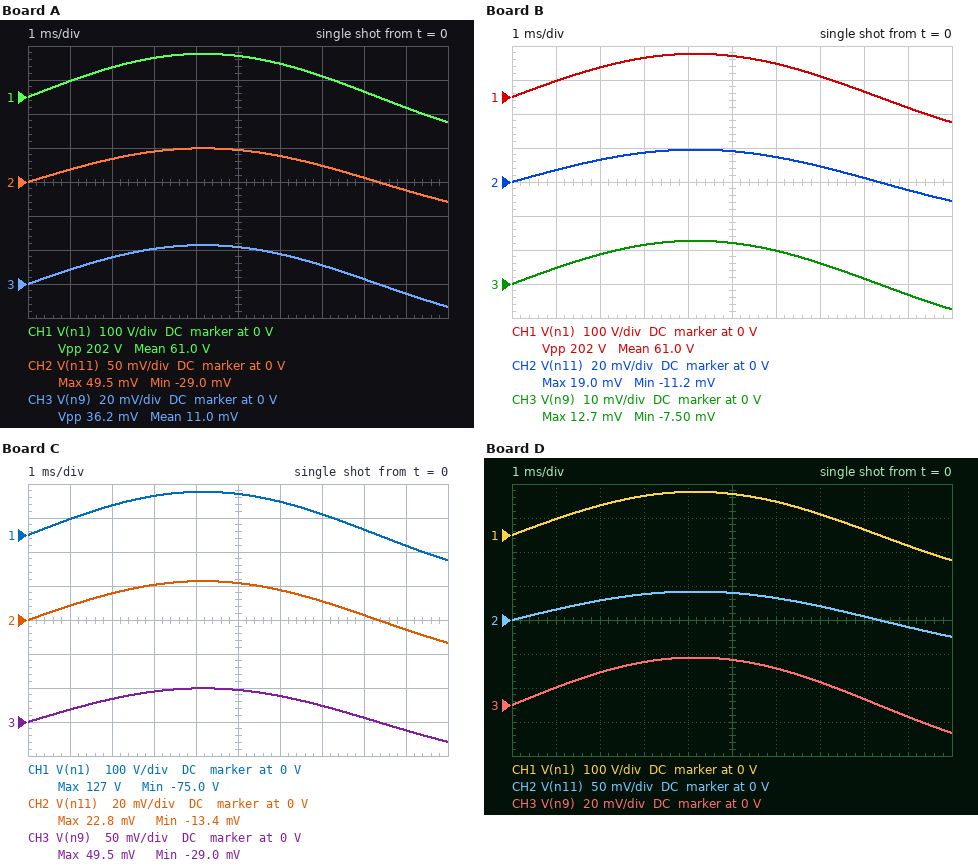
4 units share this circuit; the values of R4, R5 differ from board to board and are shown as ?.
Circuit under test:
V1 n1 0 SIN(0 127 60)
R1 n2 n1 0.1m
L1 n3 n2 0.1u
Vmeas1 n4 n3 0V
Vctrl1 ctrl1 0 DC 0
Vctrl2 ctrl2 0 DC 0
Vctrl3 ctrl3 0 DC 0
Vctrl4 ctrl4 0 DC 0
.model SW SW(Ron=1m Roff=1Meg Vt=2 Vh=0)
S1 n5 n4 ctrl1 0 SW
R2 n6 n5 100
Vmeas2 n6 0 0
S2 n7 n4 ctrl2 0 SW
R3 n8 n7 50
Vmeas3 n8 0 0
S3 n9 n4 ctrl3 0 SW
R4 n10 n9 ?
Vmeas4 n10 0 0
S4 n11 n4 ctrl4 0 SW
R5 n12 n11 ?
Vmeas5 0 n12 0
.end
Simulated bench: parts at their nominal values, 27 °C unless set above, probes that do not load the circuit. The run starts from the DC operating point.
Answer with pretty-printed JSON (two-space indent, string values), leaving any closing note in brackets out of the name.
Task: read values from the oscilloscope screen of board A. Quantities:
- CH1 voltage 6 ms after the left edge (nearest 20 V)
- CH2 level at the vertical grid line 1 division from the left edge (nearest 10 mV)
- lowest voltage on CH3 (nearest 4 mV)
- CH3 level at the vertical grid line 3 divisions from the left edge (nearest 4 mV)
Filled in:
{
  "CH1 voltage 6 ms after the left edge": "100 V",
  "CH2 level at the vertical grid line 1 division from the left edge": "20 mV",
  "lowest voltage on CH3": "-12 mV",
  "CH3 level at the vertical grid line 3 divisions from the left edge": "20 mV"
}
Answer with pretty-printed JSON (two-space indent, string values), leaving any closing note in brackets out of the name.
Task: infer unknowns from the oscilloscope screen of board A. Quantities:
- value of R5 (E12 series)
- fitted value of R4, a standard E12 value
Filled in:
{
  "value of R5": "390 Ω",
  "fitted value of R4, a standard E12 value": "180 Ω"
}
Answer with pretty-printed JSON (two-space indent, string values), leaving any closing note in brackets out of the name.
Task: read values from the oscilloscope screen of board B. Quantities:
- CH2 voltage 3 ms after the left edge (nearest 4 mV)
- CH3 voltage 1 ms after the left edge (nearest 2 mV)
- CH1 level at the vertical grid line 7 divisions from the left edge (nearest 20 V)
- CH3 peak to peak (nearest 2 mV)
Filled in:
{
  "CH2 voltage 3 ms after the left edge": "16 mV",
  "CH3 voltage 1 ms after the left edge": "4 mV",
  "CH1 level at the vertical grid line 7 divisions from the left edge": "60 V",
  "CH3 peak to peak": "20 mV"
}
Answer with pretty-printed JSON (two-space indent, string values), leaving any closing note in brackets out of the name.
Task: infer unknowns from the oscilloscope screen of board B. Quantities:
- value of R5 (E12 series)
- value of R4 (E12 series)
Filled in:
{
  "value of R5": "150 Ω",
  "value of R4": "100 Ω"
}
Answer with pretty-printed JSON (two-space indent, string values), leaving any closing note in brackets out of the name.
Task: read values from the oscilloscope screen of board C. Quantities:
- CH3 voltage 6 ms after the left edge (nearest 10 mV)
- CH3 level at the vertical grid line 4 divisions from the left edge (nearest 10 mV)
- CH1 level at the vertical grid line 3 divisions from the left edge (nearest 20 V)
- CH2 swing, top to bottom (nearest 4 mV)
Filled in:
{
  "CH3 voltage 6 ms after the left edge": "40 mV",
  "CH3 level at the vertical grid line 4 divisions from the left edge": "50 mV",
  "CH1 level at the vertical grid line 3 divisions from the left edge": "120 V",
  "CH2 swing, top to bottom": "36 mV"
}
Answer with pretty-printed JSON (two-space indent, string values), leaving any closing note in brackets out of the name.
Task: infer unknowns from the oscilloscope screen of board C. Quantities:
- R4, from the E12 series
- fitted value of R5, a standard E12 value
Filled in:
{
  "R4, from the E12 series": "390 Ω",
  "fitted value of R5, a standard E12 value": "180 Ω"
}
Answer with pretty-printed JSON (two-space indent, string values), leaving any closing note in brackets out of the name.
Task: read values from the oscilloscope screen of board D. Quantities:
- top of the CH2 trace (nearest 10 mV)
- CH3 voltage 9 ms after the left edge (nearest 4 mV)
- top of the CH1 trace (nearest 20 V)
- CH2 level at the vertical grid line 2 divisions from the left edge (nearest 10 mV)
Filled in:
{
  "top of the CH2 trace": "40 mV",
  "CH3 voltage 9 ms after the left edge": "-8 mV",
  "top of the CH1 trace": "120 V",
  "CH2 level at the vertical grid line 2 divisions from the left edge": "30 mV"
}
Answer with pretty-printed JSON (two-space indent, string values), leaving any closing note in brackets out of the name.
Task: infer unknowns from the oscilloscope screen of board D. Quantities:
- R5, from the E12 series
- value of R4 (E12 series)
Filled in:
{
  "R5, from the E12 series": "330 Ω",
  "value of R4": "220 Ω"
}
